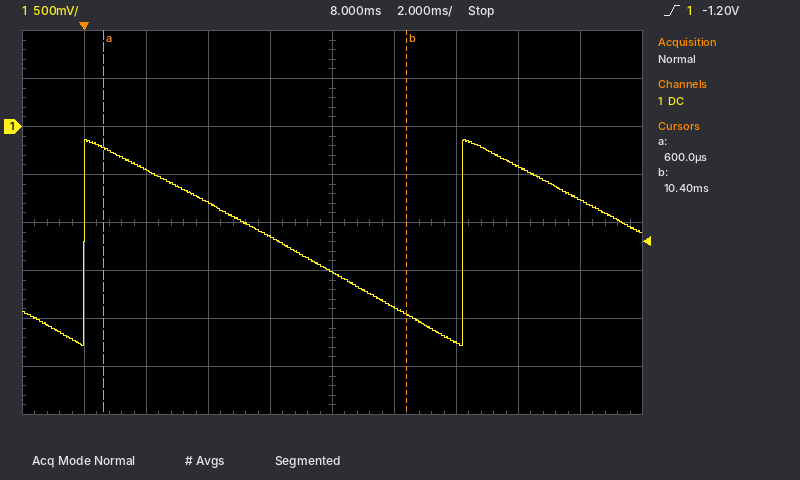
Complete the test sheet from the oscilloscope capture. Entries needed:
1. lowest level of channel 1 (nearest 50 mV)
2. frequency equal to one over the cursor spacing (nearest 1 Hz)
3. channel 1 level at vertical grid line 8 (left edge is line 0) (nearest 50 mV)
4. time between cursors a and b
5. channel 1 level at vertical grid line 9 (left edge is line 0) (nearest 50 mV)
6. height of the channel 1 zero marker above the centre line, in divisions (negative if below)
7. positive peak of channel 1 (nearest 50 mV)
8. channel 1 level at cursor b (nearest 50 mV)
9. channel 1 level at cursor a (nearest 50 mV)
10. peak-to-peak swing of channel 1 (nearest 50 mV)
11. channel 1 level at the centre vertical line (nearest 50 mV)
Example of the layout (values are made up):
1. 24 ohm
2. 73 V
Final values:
1. -2.30 V
2. 102 Hz
3. -400 mV
4. 9.8 ms
5. -750 mV
6. +2.0 div
7. -150 mV
8. -1.95 V
9. -200 mV
10. 2.15 V
11. -1.50 V
